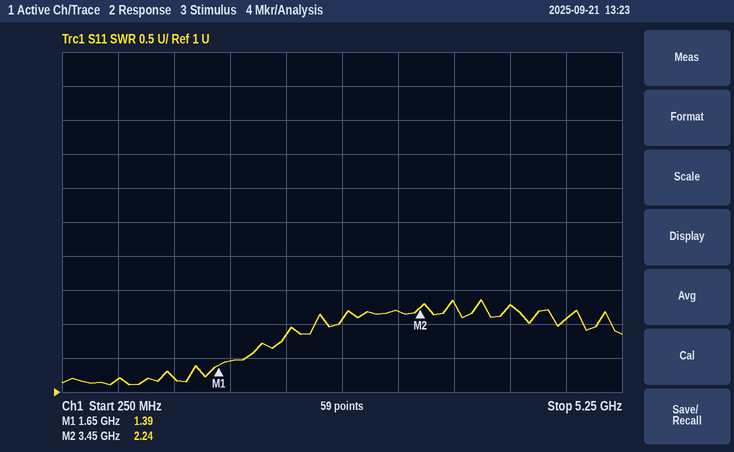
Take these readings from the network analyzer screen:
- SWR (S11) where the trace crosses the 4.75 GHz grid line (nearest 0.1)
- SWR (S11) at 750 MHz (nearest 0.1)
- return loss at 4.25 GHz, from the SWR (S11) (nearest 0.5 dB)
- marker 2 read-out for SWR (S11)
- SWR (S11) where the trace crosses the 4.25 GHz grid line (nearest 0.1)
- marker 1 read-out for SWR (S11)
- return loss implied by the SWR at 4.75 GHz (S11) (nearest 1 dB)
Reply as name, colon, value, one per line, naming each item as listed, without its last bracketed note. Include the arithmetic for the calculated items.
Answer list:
SWR (S11) where the trace crosses the 4.75 GHz grid line: 2.1
SWR (S11) at 750 MHz: 1.2
return loss at 4.25 GHz, from the SWR (S11): −20 log10((2.3 − 1)/(2.3 + 1)) ≈ 8.09 dB, so 8.0 dB to the nearest 0.5 dB
marker 2 read-out for SWR: 2.24
SWR (S11) where the trace crosses the 4.25 GHz grid line: 2.3
marker 1 read-out for SWR: 1.39
return loss implied by the SWR at 4.75 GHz (S11): −20 log10((2.1 − 1)/(2.1 + 1)) ≈ 9 dB
